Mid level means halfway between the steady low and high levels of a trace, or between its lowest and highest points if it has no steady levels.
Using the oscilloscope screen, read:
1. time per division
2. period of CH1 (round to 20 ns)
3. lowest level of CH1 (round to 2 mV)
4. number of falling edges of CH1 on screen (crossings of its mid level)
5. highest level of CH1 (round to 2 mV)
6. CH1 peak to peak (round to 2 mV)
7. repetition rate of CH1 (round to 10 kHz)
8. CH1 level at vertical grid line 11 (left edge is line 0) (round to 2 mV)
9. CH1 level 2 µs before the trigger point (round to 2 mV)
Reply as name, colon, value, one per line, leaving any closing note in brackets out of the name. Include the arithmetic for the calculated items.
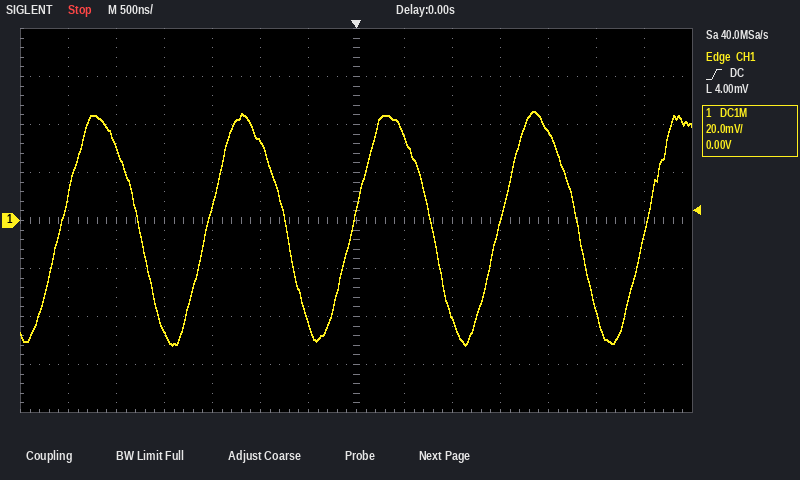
time per division: 500 ns
period of CH1: 1.52 µs
lowest level of CH1: -52 mV
number of falling edges of CH1 on screen: 4
highest level of CH1: 46 mV
CH1 peak to peak: 46 mV − (-52 mV) = 98 mV
repetition rate of CH1: 1 / 1.52 µs ≈ 658 kHz, so 660 kHz to the nearest 10 kHz
CH1 level at vertical grid line 11 (left edge is line 0): 38 mV
CH1 level 2 µs before the trigger point: -46 mV
